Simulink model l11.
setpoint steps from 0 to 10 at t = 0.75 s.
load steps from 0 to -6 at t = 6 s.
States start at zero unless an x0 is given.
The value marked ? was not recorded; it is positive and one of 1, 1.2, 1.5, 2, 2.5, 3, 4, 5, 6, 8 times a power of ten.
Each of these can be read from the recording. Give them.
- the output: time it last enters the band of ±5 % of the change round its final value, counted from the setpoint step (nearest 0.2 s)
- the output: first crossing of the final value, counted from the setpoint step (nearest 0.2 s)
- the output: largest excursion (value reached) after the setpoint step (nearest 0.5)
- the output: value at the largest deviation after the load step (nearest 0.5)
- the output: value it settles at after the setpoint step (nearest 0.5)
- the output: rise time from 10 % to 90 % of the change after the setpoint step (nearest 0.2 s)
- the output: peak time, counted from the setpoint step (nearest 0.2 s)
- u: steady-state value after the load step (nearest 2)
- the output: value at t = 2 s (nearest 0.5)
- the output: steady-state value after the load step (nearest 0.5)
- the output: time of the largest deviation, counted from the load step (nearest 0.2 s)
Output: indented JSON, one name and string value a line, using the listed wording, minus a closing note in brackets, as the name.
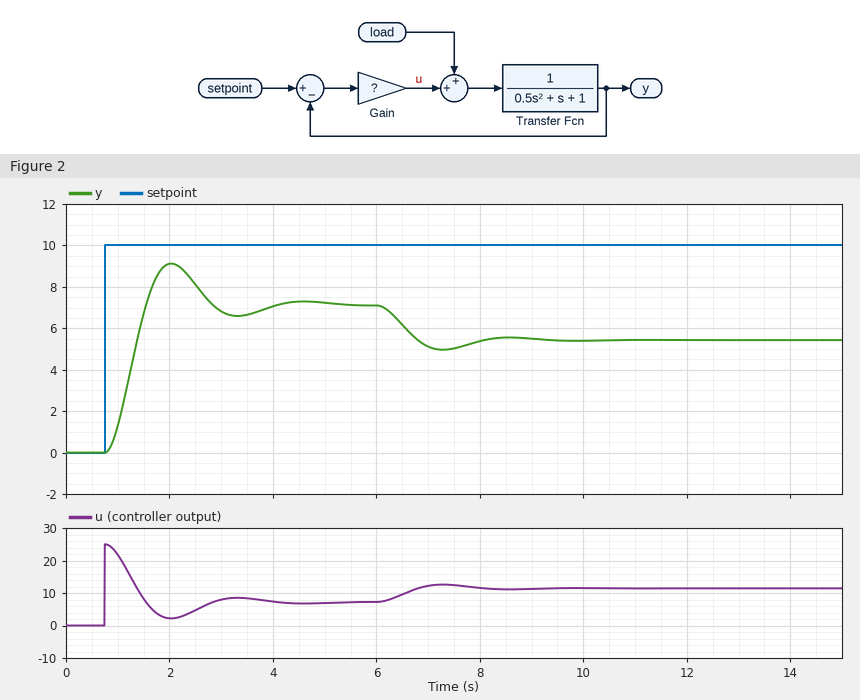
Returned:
{
  "the output: time it last enters the band of ±5 % of the change round its final value, counted from the setpoint step": "3.0 s",
  "the output: first crossing of the final value, counted from the setpoint step": "0.8 s",
  "the output: largest excursion (value reached) after the setpoint step": "9.0",
  "the output: value at the largest deviation after the load step": "5.0",
  "the output: value it settles at after the setpoint step": "7.0",
  "the output: rise time from 10 % to 90 % of the change after the setpoint step": "0.6 s",
  "the output: peak time, counted from the setpoint step": "1.2 s",
  "u: steady-state value after the load step": "12",
  "the output: value at t = 2 s": "9.0",
  "the output: steady-state value after the load step": "5.5",
  "the output: time of the largest deviation, counted from the load step": "1.2 s"
}
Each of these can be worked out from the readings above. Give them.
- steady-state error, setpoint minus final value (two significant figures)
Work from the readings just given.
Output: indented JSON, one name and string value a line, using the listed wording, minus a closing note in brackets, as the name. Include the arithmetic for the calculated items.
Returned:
{
  "steady-state error, setpoint minus final value": "10 - 7 = 3.0"
}
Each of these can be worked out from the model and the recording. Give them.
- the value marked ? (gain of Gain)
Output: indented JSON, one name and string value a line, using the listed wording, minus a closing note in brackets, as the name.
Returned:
{
  "the value marked ?": "2.5"
}
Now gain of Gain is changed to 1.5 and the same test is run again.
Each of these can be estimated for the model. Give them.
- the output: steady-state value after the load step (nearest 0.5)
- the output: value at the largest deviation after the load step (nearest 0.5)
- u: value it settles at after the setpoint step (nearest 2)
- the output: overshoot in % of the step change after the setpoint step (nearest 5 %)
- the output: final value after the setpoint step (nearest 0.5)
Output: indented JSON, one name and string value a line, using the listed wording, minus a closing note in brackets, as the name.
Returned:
{
  "the output: steady-state value after the load step": "3.5",
  "the output: value at the largest deviation after the load step": "3.0",
  "u: value it settles at after the setpoint step": "6",
  "the output: overshoot in % of the step change after the setpoint step": "20 %",
  "the output: final value after the setpoint step": "6.0"
}
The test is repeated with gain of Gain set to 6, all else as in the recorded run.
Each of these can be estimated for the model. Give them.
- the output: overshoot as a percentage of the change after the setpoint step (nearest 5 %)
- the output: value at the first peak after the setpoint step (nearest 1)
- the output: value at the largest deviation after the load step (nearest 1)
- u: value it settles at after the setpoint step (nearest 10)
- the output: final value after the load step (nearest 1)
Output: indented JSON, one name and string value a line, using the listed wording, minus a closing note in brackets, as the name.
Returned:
{
  "the output: overshoot as a percentage of the change after the setpoint step": "40 %",
  "the output: value at the first peak after the setpoint step": "12",
  "the output: value at the largest deviation after the load step": "7",
  "u: value it settles at after the setpoint step": "10",
  "the output: final value after the load step": "8"
}
